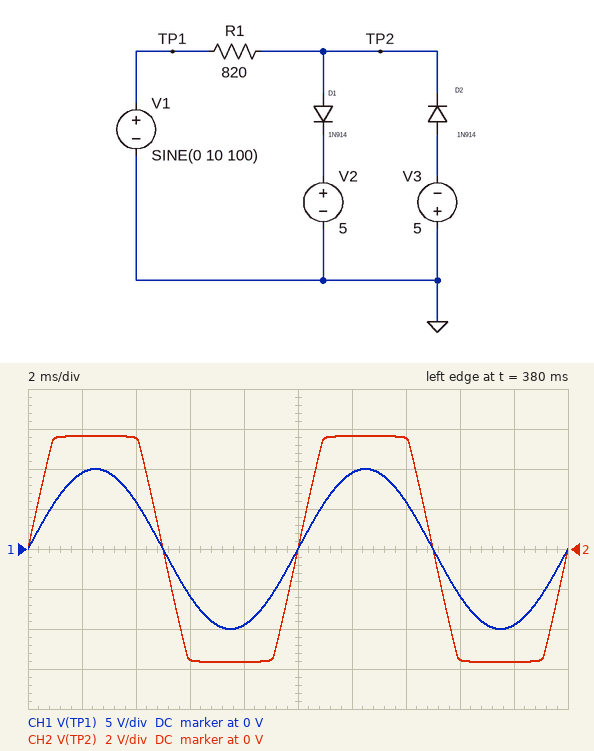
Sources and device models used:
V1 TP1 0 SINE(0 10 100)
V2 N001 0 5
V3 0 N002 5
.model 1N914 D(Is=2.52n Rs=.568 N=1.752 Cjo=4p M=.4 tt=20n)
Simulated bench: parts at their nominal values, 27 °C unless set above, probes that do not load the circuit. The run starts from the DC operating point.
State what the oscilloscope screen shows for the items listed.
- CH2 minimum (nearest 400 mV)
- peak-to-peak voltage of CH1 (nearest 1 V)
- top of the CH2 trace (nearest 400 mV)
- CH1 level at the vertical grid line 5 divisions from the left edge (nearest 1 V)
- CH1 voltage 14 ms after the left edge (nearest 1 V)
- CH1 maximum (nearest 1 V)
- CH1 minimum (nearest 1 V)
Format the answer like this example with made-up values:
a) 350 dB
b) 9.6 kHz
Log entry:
a) -5.6 V
b) 20 V
c) 5.6 V
d) 0 V
e) 6 V
f) 10 V
g) -10 V
